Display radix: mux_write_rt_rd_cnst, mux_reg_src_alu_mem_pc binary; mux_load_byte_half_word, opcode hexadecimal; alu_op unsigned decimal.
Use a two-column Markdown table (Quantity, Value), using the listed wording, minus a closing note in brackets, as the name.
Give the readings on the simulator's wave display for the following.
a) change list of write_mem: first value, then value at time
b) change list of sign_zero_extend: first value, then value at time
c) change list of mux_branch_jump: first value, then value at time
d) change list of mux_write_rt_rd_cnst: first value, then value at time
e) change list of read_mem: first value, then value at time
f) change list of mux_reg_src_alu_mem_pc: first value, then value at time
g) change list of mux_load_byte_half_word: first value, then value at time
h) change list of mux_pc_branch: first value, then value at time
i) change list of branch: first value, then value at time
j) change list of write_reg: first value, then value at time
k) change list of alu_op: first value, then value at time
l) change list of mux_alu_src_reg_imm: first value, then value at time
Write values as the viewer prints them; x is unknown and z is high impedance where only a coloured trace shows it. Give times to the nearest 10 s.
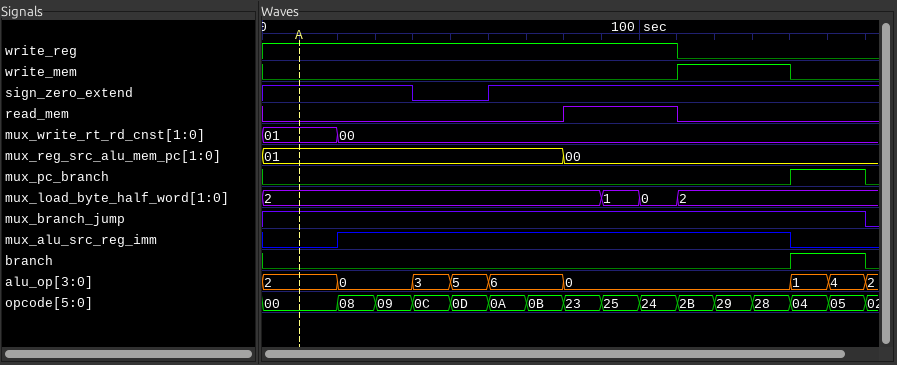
| Quantity | Value |
|---|---|
| change list of write_mem: first value, then value at time | 0, 1 at 110 s, 0 at 140 s |
| change list of sign_zero_extend: first value, then value at time | 1, 0 at 40 s, 1 at 60 s |
| change list of mux_branch_jump: first value, then value at time | 1, 0 at 160 s |
| change list of mux_write_rt_rd_cnst: first value, then value at time | 01, 00 at 20 s |
| change list of read_mem: first value, then value at time | 0, 1 at 80 s, 0 at 110 s |
| change list of mux_reg_src_alu_mem_pc: first value, then value at time | 01, 00 at 80 s |
| change list of mux_load_byte_half_word: first value, then value at time | 2, 1 at 90 s, 0 at 100 s, 2 at 110 s |
| change list of mux_pc_branch: first value, then value at time | 0, 1 at 140 s, 0 at 160 s |
| change list of branch: first value, then value at time | 0, 1 at 140 s, 0 at 160 s |
| change list of write_reg: first value, then value at time | 1, 0 at 110 s |
| change list of alu_op: first value, then value at time | 2, 0 at 20 s, 3 at 40 s, 5 at 50 s, 6 at 60 s, 0 at 80 s, 1 at 140 s, 4 at 150 s, 2 at 160 s |
| change list of mux_alu_src_reg_imm: first value, then value at time | 0, 1 at 20 s, 0 at 140 s |
